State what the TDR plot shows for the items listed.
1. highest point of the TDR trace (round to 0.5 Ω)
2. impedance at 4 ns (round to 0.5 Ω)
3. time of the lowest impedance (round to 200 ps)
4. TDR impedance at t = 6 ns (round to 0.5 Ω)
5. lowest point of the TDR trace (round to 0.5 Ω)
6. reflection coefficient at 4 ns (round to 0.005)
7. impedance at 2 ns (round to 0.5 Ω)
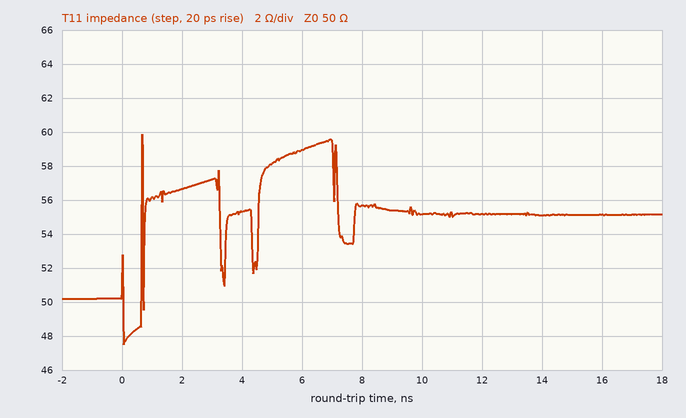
60.0 Ω
55.5 Ω
0.0 ns
59.0 Ω
47.5 Ω
+0.050
56.5 Ω
